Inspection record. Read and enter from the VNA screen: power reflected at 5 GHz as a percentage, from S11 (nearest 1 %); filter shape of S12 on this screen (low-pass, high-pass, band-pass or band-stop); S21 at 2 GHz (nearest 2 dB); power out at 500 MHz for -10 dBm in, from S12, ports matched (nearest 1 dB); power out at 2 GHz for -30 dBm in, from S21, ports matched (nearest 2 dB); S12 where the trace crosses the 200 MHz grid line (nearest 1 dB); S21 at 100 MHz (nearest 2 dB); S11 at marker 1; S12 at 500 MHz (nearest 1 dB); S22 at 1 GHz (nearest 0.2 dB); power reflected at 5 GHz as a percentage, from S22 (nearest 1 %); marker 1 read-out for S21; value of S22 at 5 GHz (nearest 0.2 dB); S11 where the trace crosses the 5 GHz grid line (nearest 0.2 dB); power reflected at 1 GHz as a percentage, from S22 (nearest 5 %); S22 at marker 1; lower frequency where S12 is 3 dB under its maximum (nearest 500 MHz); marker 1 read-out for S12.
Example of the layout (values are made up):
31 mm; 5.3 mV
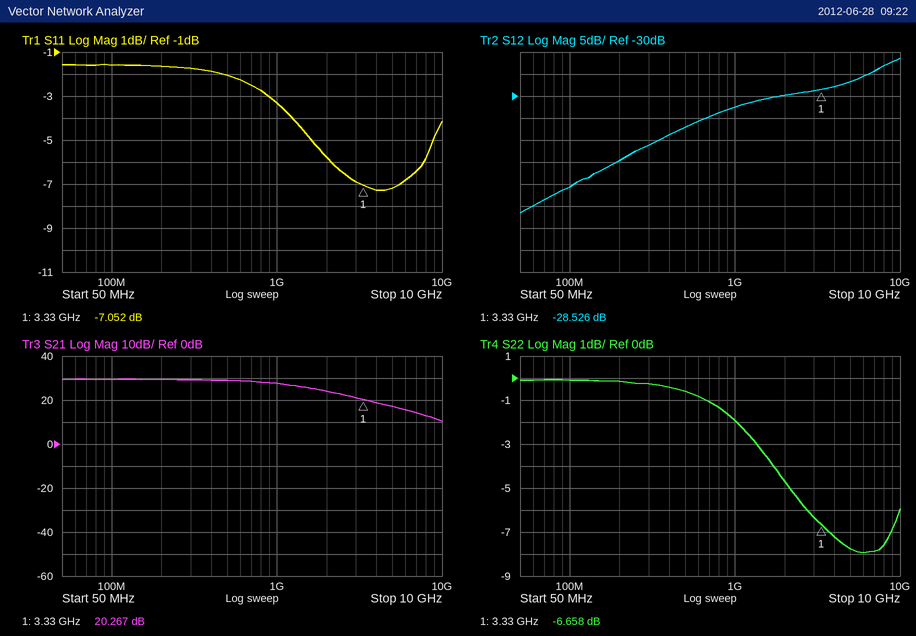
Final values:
19 %; high-pass; 24 dB; -47 dBm; -6 dBm; -45 dB; 30 dB; -7.052 dB; -37 dB; -2.0 dB; 17 %; 20.267 dB; -7.8 dB; -7.2 dB; 65 %; -6.658 dB; 7.0 GHz; -28.526 dB
